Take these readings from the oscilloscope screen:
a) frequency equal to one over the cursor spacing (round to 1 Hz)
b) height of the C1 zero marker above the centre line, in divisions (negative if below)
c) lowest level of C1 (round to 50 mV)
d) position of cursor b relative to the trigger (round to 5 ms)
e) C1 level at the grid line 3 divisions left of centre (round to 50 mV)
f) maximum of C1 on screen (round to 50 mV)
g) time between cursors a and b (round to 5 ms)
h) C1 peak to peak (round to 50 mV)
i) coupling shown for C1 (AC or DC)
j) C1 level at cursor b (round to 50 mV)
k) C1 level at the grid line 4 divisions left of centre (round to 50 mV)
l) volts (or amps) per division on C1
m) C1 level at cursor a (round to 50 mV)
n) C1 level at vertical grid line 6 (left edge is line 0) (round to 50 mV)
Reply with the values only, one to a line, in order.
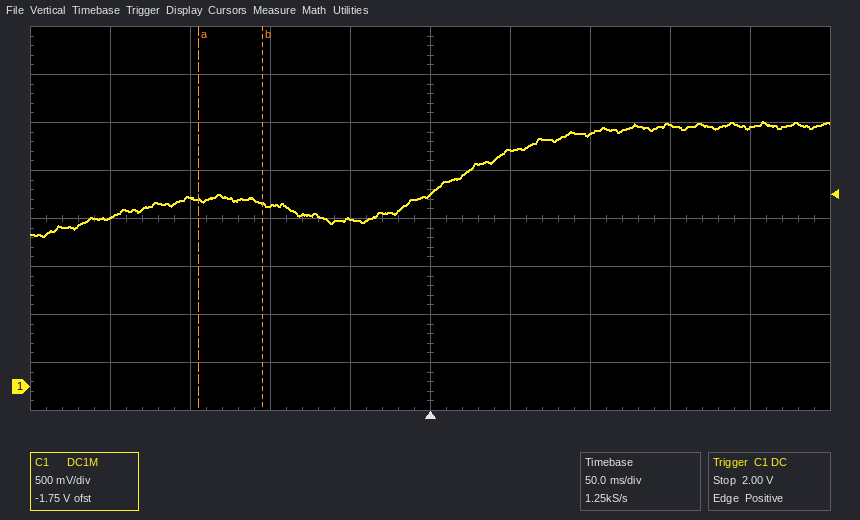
25 Hz
-3.5 div
1.55 V
-105 ms
1.95 V
2.75 V
40 ms
1.20 V
DC
1.90 V
1.75 V
500 mV
1.95 V
2.45 V
